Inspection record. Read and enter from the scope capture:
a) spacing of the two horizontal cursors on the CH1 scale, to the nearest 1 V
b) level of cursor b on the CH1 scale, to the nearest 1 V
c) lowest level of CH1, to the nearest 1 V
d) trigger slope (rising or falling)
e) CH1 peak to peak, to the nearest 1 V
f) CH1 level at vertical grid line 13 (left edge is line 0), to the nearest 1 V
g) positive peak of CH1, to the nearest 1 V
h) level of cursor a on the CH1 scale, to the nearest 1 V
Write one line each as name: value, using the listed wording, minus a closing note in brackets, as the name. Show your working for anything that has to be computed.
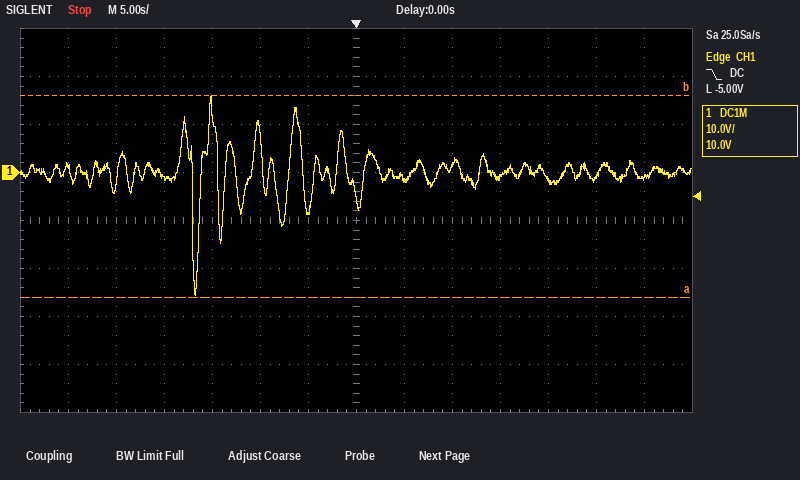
spacing of the two horizontal cursors on the CH1 scale, to the nearest 1 V: 42 V
level of cursor b on the CH1 scale, to the nearest 1 V: 16 V
lowest level of CH1, to the nearest 1 V: -26 V
trigger slope: falling
CH1 peak to peak, to the nearest 1 V: 16 V − (-26 V) = 42 V
CH1 level at vertical grid line 13 (left edge is line 0), to the nearest 1 V: -1 V
positive peak of CH1, to the nearest 1 V: 16 V
level of cursor a on the CH1 scale, to the nearest 1 V: -26 V
